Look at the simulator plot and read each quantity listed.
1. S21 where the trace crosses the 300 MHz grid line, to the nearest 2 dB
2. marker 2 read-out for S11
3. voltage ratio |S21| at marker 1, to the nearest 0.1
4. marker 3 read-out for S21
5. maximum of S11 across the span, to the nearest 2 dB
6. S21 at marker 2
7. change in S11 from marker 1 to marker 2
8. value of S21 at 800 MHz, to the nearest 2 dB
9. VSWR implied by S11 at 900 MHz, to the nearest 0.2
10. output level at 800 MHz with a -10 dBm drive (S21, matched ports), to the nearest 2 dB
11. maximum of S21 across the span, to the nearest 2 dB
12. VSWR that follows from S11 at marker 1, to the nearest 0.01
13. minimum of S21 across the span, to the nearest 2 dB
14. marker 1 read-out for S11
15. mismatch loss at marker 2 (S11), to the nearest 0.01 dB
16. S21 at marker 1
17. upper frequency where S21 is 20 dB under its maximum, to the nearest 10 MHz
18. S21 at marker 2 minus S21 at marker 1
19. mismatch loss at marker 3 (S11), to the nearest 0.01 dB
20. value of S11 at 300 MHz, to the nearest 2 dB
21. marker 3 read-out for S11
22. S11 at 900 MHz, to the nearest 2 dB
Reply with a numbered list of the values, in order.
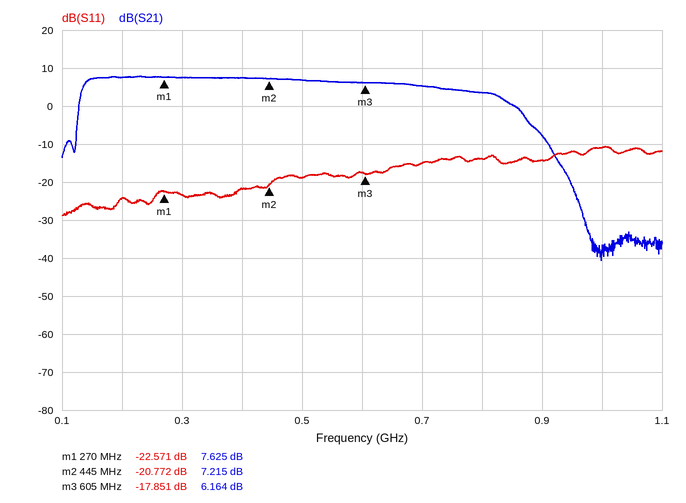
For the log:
1. 8 dB
2. -20.772 dB
3. 2.4
4. 6.164 dB
5. -10 dB
6. 7.215 dB
7. 1.799 dB
8. 4 dB
9. 1.4
10. -6 dBm
11. 8 dB
12. 1.16
13. -40 dB
14. -22.571 dB
15. 0.04 dB
16. 7.625 dB
17. 920 MHz
18. -0.410 dB
19. 0.07 dB
20. -24 dB
21. -17.851 dB
22. -14 dB
